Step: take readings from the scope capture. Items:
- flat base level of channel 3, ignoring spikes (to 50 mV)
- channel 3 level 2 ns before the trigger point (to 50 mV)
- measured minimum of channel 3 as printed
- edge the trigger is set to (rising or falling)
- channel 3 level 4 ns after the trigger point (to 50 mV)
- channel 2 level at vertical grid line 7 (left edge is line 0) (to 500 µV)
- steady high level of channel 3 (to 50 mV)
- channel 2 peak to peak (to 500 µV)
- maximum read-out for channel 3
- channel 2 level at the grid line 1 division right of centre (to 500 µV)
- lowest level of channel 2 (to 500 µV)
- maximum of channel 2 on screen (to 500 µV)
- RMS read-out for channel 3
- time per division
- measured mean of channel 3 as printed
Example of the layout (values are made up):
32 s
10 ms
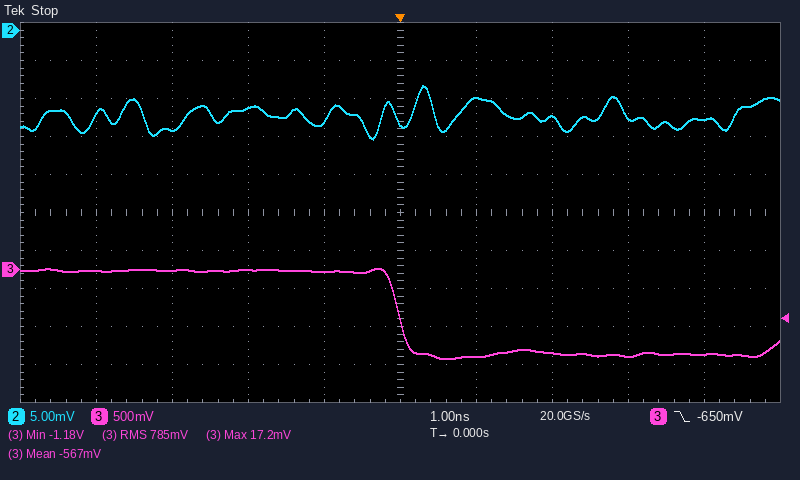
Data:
-1.10 V
0 mV
-1.18 V
falling
-1.10 V
-11.5 mV
0 mV
7.0 mV
17.2 mV
-9.0 mV
-14.5 mV
-7.5 mV
785 mV
1 ns
-567 mV
